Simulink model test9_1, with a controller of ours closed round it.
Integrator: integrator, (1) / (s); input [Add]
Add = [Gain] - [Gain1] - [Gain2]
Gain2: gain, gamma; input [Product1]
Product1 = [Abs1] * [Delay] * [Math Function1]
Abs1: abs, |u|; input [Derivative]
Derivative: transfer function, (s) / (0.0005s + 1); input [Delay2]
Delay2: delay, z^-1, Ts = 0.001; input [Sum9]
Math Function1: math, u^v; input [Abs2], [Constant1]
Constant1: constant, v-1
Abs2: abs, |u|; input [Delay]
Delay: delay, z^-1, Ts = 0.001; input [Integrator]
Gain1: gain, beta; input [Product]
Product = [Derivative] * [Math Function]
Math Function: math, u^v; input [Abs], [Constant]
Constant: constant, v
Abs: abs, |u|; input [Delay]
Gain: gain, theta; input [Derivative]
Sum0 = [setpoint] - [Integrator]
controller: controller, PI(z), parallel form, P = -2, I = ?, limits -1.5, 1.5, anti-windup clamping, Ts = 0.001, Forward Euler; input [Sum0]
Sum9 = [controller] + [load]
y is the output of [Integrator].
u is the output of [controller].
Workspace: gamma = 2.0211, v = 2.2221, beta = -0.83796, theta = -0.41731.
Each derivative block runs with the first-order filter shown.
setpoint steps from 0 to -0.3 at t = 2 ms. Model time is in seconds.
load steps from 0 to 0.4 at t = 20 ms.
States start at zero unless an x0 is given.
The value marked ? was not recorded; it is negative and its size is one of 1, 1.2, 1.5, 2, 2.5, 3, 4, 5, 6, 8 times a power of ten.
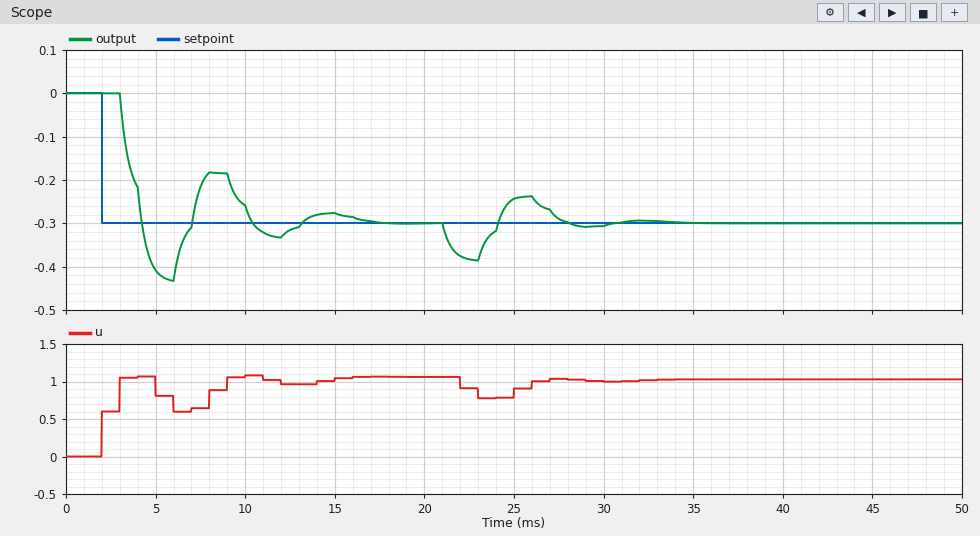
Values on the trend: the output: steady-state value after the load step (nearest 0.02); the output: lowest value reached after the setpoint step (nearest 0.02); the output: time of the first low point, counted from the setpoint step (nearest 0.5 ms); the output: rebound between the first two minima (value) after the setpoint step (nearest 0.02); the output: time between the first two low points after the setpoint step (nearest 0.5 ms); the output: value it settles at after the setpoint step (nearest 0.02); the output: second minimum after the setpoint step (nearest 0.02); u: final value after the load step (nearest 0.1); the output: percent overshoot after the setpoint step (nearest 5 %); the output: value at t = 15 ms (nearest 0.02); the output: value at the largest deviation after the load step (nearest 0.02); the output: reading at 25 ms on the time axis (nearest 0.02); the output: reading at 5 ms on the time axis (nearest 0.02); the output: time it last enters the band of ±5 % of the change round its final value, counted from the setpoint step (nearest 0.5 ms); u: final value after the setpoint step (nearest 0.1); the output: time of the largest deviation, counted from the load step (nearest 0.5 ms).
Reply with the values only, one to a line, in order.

-0.30
-0.44
4.0 ms
-0.18
6.0 ms
-0.30
-0.34
1.0
45 %
-0.28
-0.38
-0.24
-0.40
14.0 ms
1.1
3.0 ms
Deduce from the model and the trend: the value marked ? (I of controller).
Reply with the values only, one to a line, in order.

-1500
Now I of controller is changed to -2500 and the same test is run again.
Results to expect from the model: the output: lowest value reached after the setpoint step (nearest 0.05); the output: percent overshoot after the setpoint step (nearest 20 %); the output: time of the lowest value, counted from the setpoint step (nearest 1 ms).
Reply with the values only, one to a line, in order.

-0.60
120 %
4 ms
